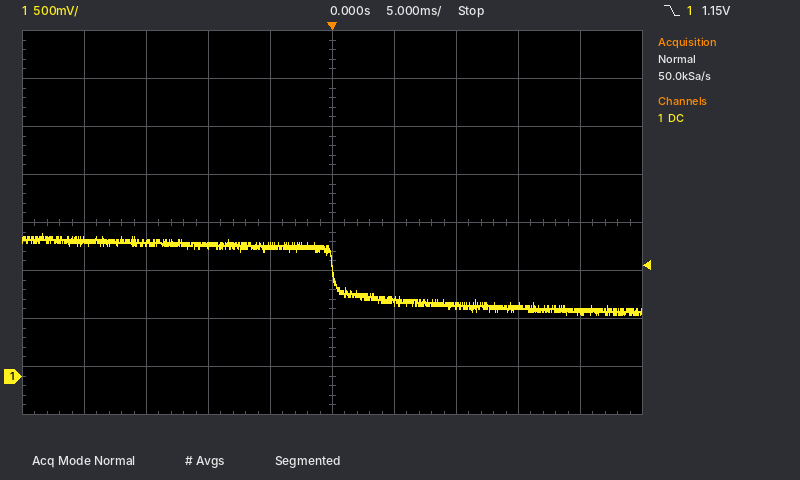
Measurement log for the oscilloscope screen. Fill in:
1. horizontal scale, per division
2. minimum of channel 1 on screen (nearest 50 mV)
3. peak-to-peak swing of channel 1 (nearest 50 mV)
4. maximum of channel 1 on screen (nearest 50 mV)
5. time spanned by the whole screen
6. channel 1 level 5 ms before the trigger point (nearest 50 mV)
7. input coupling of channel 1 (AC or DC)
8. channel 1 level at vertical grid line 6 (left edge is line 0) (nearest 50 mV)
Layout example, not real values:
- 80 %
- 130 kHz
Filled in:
- 5 ms
- 650 mV
- 850 mV
- 1.50 V
- 50 ms
- 1.35 V
- DC
- 800 mV
